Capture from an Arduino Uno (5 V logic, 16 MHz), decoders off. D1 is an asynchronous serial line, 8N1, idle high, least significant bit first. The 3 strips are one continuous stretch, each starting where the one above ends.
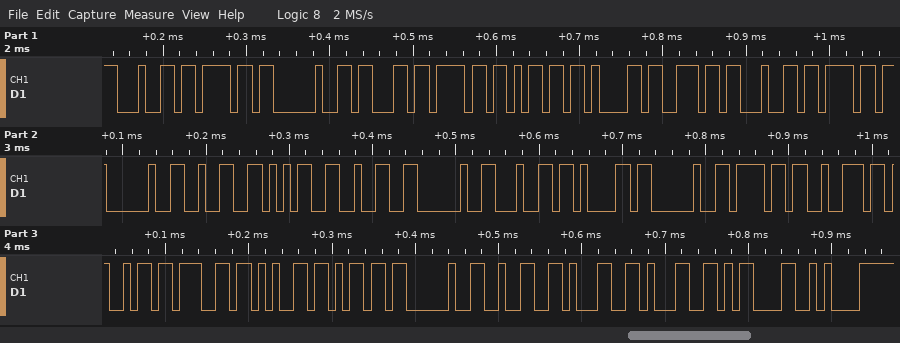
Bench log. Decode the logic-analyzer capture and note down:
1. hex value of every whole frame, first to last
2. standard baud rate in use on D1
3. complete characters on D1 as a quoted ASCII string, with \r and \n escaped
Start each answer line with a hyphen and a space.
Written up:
- 64 6F 20 63 6F 6D 61 6E 64 6F 20 32 35 32 20 64 61 20 6F 72 69 67 65 6D 20 32 31 31 0D 0A
- 115200 baud
- "do comando 252 da origem 211\r\n"
